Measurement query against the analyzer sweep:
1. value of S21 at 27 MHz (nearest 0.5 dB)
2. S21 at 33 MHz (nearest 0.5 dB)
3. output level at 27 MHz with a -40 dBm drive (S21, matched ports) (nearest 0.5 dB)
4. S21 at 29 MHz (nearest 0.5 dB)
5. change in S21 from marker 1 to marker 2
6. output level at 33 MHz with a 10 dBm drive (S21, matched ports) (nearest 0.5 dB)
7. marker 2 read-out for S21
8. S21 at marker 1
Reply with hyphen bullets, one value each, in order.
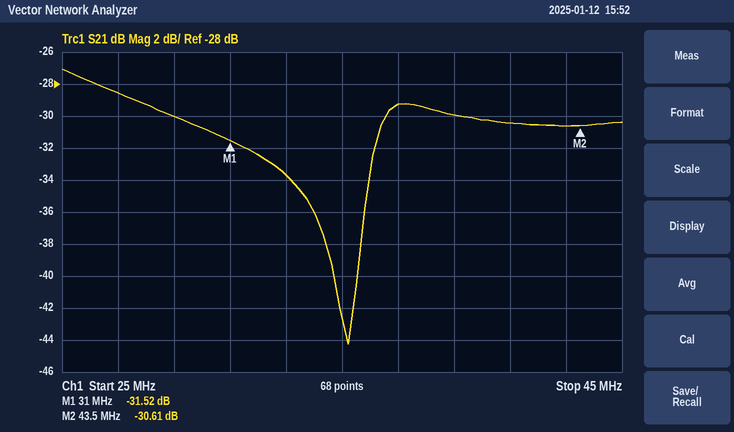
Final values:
- -28.5 dB
- -33.5 dB
- -68.5 dBm
- -30.0 dB
- 0.91 dB
- -23.5 dBm
- -30.61 dB
- -31.52 dB
